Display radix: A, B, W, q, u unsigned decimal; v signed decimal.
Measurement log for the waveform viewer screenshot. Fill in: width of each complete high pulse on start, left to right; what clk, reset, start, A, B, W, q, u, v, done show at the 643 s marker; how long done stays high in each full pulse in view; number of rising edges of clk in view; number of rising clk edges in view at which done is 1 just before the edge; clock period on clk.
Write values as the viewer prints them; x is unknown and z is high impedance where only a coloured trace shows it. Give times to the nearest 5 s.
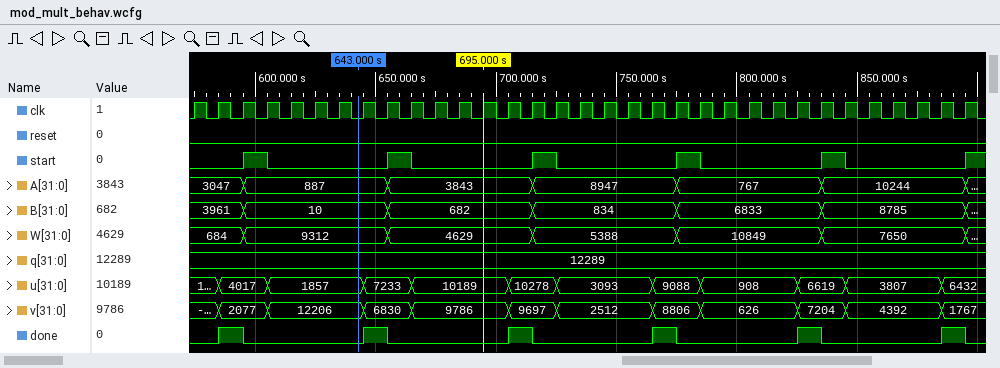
10 s, 10 s, 10 s, 10 s, 10 s
clk=0, reset=0, start=0, A=887, B=10, W=9312, q=12289, u=1857, v=12206, done=0
10 s, 10 s, 10 s, 10 s, 10 s, 10 s
33
6
10 s
